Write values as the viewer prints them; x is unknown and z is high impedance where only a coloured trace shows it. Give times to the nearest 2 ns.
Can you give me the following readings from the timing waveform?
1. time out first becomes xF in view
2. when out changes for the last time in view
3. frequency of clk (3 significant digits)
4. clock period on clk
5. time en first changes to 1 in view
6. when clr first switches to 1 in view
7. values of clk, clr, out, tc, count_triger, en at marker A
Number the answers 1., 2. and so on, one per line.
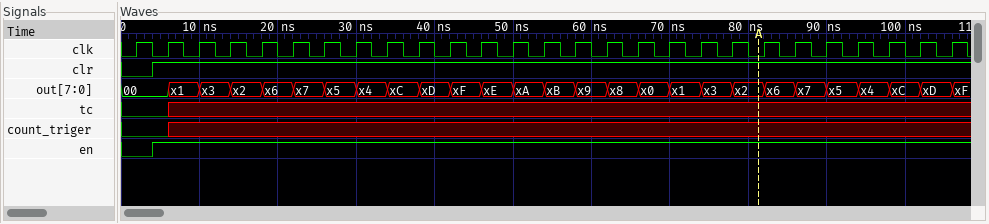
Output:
1. 42 ns
2. 106 ns
3. 250 MHz
4. 4 ns
5. 4 ns
6. 4 ns
7. clk=0, clr=1, out=x2, tc=x, count_triger=x, en=1
